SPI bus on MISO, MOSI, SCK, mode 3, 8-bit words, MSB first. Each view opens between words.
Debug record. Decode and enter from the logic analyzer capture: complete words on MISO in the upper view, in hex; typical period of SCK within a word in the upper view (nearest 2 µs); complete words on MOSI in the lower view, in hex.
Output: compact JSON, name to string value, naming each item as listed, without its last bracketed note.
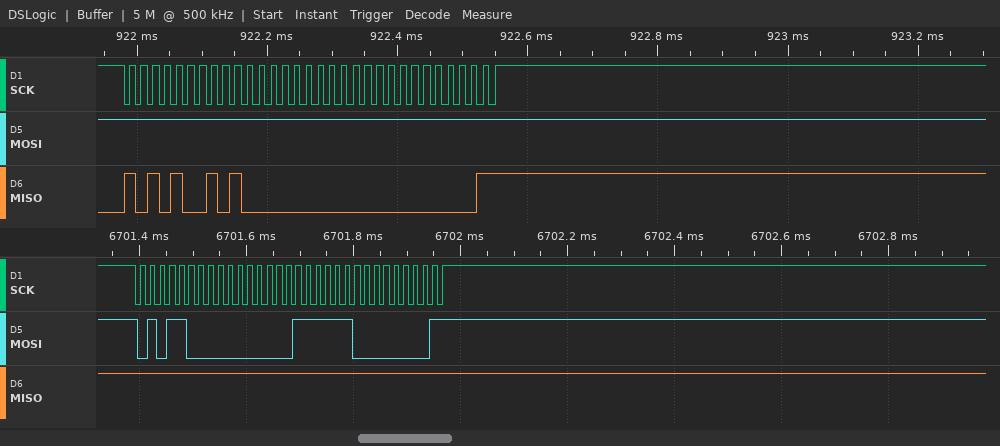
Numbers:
{"complete words on MISO in the upper view, in hex": "A9, 40, 00, 03", "typical period of SCK within a word in the upper view": "18 µs", "complete words on MOSI in the lower view, in hex": "58, 00, FC, 03"}
